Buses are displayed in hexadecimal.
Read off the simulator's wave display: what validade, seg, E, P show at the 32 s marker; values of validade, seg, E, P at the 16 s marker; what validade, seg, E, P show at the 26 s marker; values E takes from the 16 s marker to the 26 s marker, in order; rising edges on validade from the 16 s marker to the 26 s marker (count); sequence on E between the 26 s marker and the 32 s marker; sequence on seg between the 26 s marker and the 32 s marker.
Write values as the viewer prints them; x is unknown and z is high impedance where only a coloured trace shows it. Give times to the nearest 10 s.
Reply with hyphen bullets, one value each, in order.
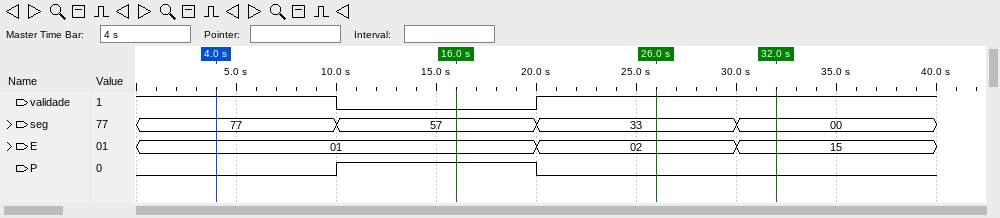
- validade=1, seg=00, E=15, P=0
- validade=0, seg=57, E=01, P=1
- validade=1, seg=33, E=02, P=0
- 01, 02
- 1
- 02, 15
- 33, 00
